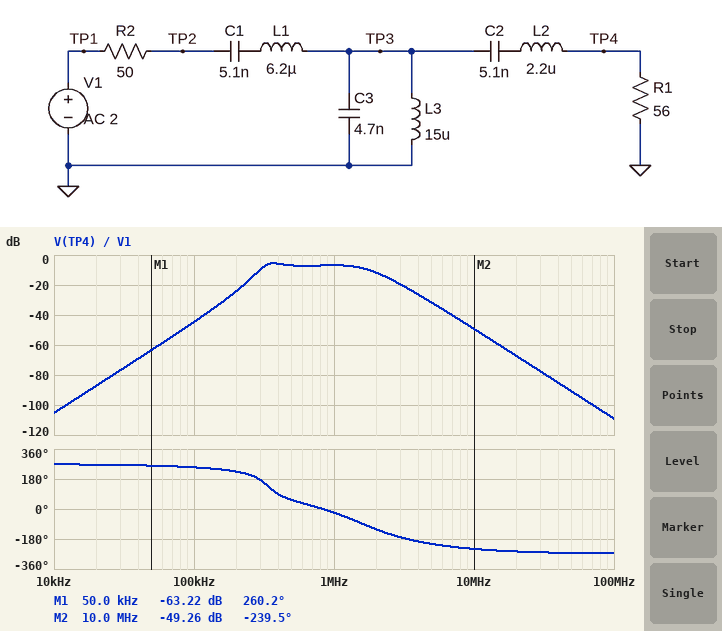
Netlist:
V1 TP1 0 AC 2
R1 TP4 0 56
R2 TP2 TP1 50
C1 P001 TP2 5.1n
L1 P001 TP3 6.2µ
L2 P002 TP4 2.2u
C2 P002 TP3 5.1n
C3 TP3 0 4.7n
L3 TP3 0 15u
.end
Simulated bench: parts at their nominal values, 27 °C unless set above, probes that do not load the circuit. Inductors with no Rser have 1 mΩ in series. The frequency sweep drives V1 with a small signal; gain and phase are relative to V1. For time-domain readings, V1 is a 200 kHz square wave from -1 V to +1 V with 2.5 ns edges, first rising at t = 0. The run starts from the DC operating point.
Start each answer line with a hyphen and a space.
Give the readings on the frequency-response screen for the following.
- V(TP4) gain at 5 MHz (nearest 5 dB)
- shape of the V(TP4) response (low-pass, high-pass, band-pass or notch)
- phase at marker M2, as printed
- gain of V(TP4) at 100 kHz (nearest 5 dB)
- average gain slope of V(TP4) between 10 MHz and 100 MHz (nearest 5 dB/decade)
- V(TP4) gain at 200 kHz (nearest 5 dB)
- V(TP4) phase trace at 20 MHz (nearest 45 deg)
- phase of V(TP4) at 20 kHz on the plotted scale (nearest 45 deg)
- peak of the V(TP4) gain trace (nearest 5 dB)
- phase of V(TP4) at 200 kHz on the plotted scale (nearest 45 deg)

- -30 dB
- band-pass
- -239.5 deg
- -45 dB
- -60 dB/decade
- -25 dB
- -270 deg
- 270 deg
- -5 dB
- 225 deg
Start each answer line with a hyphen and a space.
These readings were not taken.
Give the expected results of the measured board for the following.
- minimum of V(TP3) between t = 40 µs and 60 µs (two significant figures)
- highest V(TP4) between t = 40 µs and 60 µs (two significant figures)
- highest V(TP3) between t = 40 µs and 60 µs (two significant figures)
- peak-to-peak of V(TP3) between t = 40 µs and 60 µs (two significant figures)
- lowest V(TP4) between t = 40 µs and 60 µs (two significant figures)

- -470 mV
- 380 mV
- 470 mV
- 940 mV
- -380 mV
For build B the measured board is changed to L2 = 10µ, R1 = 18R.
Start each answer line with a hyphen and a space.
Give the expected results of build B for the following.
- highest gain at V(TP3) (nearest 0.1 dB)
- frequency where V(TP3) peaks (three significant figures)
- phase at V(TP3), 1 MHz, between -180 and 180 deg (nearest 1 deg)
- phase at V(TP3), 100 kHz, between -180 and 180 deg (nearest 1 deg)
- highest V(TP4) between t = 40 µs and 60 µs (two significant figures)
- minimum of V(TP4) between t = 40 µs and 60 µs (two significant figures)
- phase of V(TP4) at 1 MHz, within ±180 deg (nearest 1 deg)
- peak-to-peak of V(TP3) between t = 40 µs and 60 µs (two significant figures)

- 1.7 dB
- 327 kHz
- 5 deg
- 170 deg
- 190 mV
- -190 mV
- -56 deg
- 1.0 V
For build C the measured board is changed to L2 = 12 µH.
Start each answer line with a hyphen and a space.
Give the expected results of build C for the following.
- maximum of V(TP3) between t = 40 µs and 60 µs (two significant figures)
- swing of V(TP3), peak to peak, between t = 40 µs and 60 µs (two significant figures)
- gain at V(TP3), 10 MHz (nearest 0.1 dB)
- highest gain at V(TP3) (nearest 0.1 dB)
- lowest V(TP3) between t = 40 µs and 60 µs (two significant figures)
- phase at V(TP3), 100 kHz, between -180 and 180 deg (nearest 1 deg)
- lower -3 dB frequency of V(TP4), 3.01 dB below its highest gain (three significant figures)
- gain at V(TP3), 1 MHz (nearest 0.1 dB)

- 590 mV
- 1.2 V
- -41.1 dB
- -2.1 dB
- -590 mV
- 170 deg
- 298 kHz
- -4.0 dB
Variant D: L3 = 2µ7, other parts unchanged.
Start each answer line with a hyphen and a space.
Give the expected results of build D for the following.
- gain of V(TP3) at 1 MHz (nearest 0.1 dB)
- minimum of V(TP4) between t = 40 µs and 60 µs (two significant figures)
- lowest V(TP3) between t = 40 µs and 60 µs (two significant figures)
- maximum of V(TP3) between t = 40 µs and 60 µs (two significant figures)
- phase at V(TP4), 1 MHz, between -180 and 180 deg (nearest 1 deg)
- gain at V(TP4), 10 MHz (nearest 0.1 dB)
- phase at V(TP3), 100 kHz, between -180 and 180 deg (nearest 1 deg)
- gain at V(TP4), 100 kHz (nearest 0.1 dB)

- -7.2 dB
- -360 mV
- -410 mV
- 410 mV
- 46 deg
- -49.1 dB
- 171 deg
- -60.2 dB
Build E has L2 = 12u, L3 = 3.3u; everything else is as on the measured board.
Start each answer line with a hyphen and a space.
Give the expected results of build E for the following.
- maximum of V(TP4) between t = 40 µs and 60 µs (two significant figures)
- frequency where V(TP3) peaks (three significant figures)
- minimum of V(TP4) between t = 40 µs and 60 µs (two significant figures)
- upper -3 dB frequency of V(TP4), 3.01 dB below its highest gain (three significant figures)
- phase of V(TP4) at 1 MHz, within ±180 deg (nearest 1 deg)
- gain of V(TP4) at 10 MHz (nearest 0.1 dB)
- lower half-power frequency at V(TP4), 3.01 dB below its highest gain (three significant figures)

- 320 mV
- 1.66 MHz
- -320 mV
- 1.85 MHz
- -2 deg
- -63.5 dB
- 707 kHz
